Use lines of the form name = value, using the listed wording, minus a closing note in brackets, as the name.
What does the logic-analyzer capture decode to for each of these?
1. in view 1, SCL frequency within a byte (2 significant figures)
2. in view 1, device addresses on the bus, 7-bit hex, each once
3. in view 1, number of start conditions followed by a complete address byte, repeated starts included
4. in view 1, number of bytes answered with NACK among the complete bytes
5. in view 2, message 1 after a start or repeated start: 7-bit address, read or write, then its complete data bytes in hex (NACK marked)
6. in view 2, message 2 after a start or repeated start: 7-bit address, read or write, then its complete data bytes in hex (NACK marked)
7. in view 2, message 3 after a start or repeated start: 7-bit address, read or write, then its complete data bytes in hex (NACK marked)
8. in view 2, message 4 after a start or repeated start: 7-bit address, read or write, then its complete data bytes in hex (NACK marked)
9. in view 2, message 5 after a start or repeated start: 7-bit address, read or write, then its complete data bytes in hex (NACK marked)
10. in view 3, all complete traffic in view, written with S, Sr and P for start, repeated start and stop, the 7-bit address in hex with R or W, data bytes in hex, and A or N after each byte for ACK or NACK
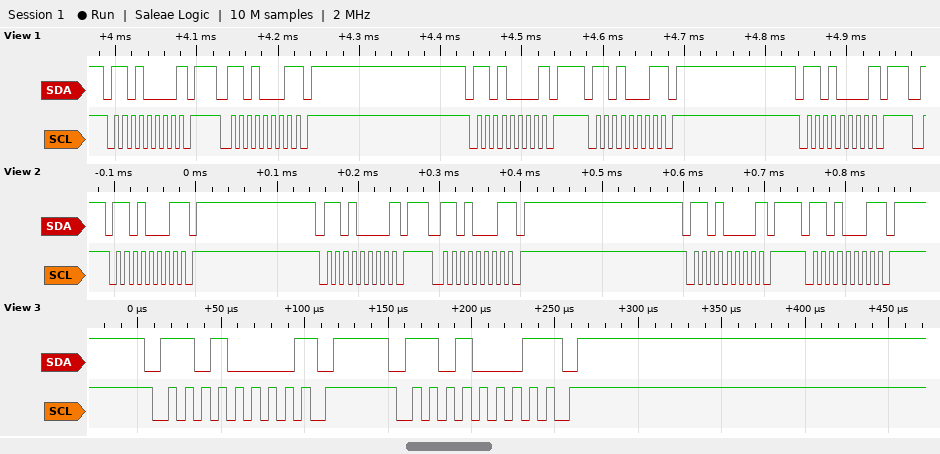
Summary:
in view 1, SCL frequency within a byte = 100 kHz
in view 1, device addresses on the bus, 7-bit hex, each once = 0x68
in view 1, number of start conditions followed by a complete address byte, repeated starts included = 5
in view 1, number of bytes answered with NACK among the complete bytes = 5
in view 2, message 1 after a start or repeated start: 7-bit address, read or write, then its complete data bytes in hex = 0x68 read NACK
in view 2, message 2 after a start or repeated start: 7-bit address, read or write, then its complete data bytes in hex = 0x68 write NACK
in view 2, message 3 after a start or repeated start: 7-bit address, read or write, then its complete data bytes in hex = 0x68 read NACK
in view 2, message 4 after a start or repeated start: 7-bit address, read or write, then its complete data bytes in hex = 0x68 write NACK
in view 2, message 5 after a start or repeated start: 7-bit address, read or write, then its complete data bytes in hex = 0x68 read NACK
in view 3, all complete traffic in view, written with S, Sr and P for start, repeated start and stop, the 7-bit address in hex with R or W, data bytes in hex, and A or N after each byte for ACK or NACK = S 68W N P S 68R N P
